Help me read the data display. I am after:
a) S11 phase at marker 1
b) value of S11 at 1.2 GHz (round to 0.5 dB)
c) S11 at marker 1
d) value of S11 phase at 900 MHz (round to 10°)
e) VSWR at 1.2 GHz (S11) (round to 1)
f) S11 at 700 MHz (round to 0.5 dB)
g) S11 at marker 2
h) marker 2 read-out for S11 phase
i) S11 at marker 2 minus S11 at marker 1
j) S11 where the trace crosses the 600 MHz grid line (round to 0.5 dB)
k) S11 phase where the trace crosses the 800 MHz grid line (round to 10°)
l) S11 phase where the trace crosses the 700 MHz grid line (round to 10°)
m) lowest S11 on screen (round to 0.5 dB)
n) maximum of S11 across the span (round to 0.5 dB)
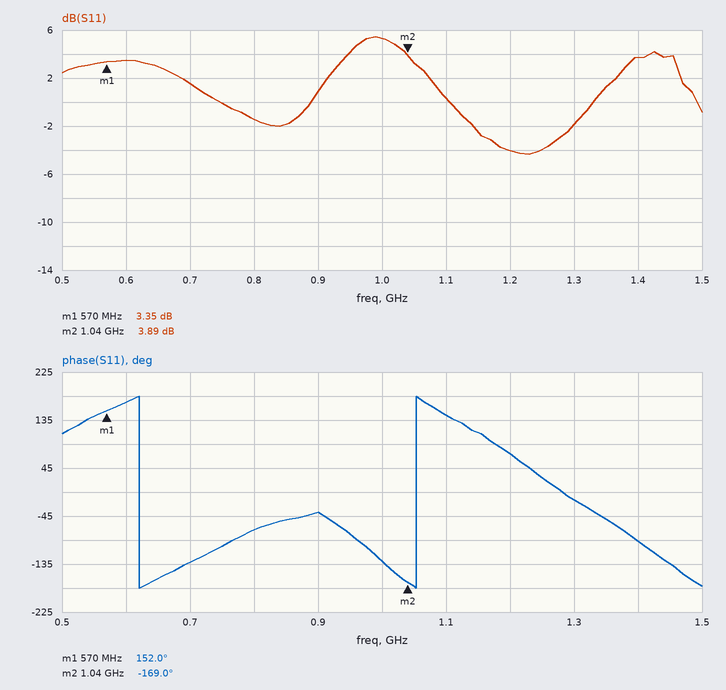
152.0°
-4.0 dB
3.35 dB
-40°
4
1.5 dB
3.89 dB
-169.0°
0.54 dB
3.5 dB
-70°
-130°
-4.5 dB
5.5 dB
